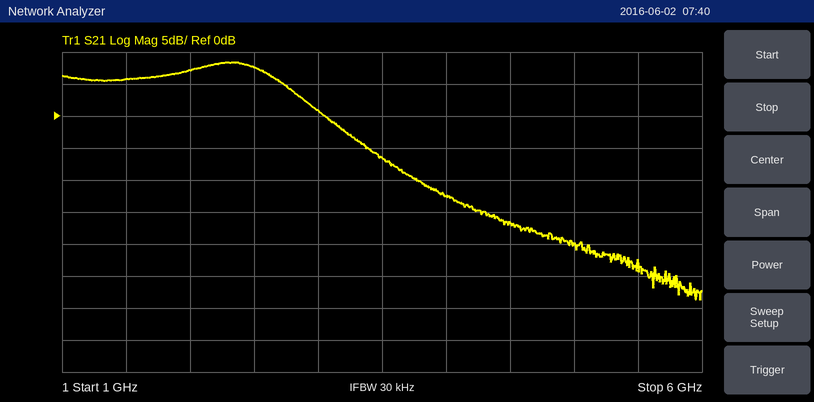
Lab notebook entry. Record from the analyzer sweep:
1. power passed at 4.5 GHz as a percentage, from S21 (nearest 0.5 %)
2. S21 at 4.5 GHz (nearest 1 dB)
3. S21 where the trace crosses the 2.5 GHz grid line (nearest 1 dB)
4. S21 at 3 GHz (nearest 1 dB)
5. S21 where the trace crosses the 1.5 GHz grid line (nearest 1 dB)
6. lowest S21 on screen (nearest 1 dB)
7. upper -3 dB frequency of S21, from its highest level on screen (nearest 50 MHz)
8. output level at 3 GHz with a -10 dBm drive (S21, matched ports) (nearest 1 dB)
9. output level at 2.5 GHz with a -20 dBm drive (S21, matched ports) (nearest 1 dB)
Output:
2.0 %
-17 dB
8 dB
1 dB
6 dB
-29 dB
2.70 GHz
-9 dBm
-12 dBm
